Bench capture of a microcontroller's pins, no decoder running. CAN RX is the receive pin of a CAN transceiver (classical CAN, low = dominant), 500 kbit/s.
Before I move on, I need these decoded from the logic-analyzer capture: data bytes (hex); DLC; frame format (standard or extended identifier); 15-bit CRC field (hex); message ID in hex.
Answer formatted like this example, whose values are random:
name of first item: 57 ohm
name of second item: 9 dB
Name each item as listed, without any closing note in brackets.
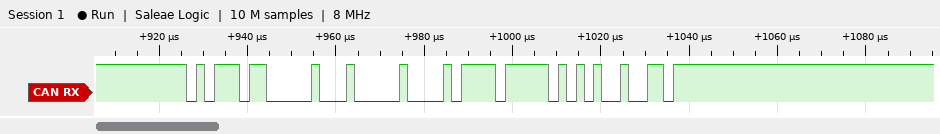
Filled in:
data bytes: 00 BD
DLC: 2
frame format: standard
15-bit CRC field: 0x7D49
message ID in hex: 0x5D8
